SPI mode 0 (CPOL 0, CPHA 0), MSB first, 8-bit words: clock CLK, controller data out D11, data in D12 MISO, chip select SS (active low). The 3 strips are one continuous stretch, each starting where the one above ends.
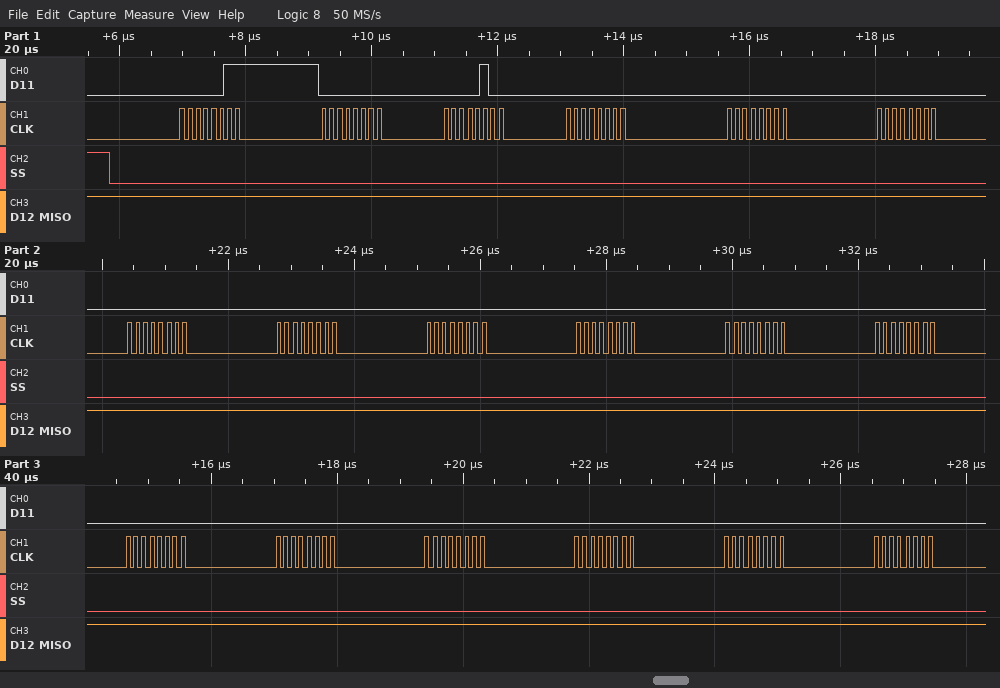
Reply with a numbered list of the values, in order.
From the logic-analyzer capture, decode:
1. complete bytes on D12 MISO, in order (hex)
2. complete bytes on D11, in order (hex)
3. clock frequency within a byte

1. 0xFF 0xFF 0xFF 0xFF 0xFF 0xFF 0xFF 0xFF 0xFF 0xFF 0xFF 0xFF 0xFF 0xFF 0xFF 0xFF 0xFF 0xFF
2. 0x03 0x00 0x04 0x00 0x00 0x00 0x00 0x00 0x00 0x00 0x00 0x00 0x00 0x00 0x00 0x00 0x00 0x00
3. 8 MHz
